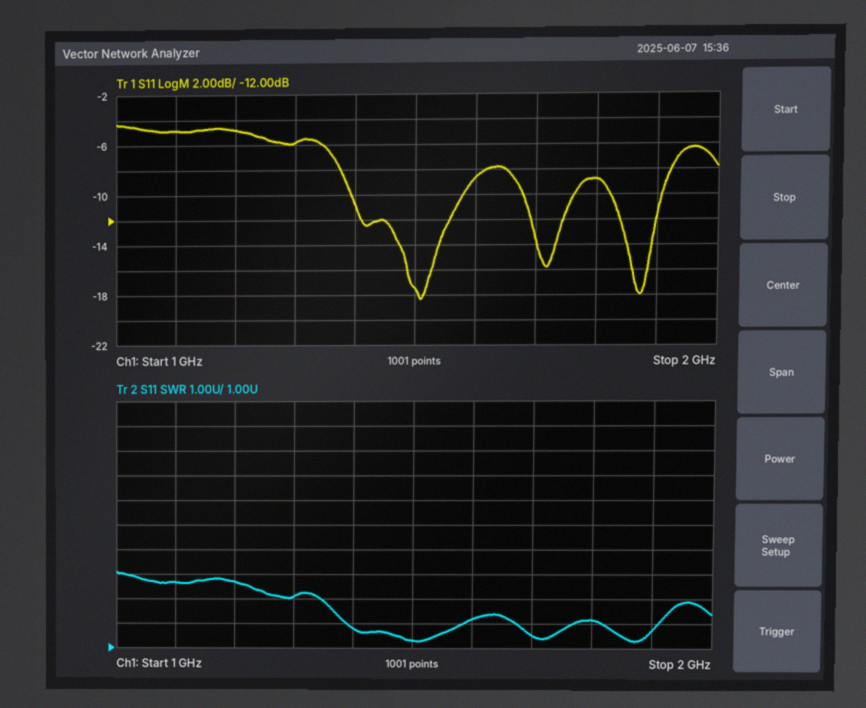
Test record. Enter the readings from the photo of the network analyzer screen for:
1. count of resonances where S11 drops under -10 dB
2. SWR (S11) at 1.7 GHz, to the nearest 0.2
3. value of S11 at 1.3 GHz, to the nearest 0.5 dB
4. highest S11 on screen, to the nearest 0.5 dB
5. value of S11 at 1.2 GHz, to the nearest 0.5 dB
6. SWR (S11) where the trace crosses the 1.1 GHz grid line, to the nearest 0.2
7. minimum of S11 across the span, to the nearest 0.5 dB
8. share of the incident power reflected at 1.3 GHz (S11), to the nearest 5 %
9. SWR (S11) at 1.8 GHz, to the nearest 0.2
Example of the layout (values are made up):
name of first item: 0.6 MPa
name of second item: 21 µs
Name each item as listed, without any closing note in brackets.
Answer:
count of resonances where S11 drops under -10 dB: 3
SWR (S11) at 1.7 GHz, to the nearest 0.2: 1.6
value of S11 at 1.3 GHz, to the nearest 0.5 dB: -6.0 dB
highest S11 on screen, to the nearest 0.5 dB: -4.5 dB
value of S11 at 1.2 GHz, to the nearest 0.5 dB: -5.0 dB
SWR (S11) where the trace crosses the 1.1 GHz grid line, to the nearest 0.2: 3.6
minimum of S11 across the span, to the nearest 0.5 dB: -18.5 dB
share of the incident power reflected at 1.3 GHz (S11), to the nearest 5 %: 25 %
SWR (S11) at 1.8 GHz, to the nearest 0.2: 2.2
